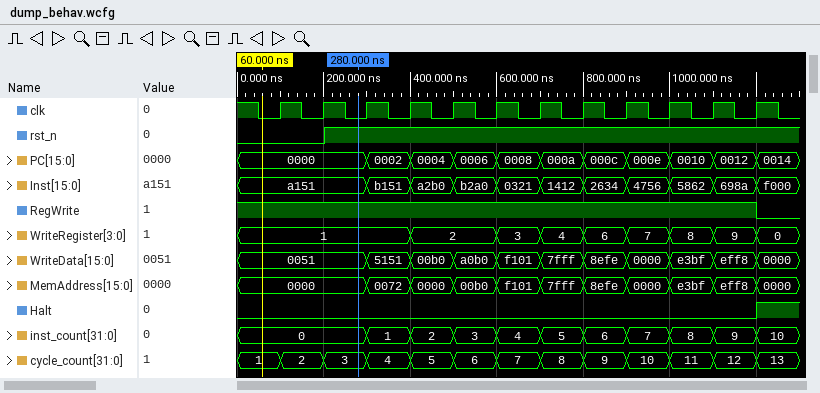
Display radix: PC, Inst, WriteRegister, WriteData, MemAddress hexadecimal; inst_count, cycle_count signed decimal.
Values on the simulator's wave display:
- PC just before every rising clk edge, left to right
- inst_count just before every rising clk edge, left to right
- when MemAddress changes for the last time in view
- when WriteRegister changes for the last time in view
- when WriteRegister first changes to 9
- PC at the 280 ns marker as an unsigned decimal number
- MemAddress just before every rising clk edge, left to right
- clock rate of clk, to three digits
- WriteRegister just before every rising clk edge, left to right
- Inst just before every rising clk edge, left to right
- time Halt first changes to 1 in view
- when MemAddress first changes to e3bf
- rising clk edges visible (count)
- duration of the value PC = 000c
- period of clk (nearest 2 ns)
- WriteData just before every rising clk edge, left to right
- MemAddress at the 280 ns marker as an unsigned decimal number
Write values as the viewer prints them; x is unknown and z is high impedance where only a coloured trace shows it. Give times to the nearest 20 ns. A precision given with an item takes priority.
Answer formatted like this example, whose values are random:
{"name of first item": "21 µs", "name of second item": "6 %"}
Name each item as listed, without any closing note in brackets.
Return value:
{"PC just before every rising clk edge, left to right": "0000, 0000, 0000, 0002, 0004, 0006, 0008, 000a, 000c, 000e, 0010, 0012", "inst_count just before every rising clk edge, left to right": "0, 0, 0, 1, 2, 3, 4, 5, 6, 7, 8, 9", "when MemAddress changes for the last time in view": "1200 ns", "when WriteRegister changes for the last time in view": "1200 ns", "when WriteRegister first changes to 9": "1100 ns", "PC at the 280 ns marker as an unsigned decimal number": "0", "MemAddress just before every rising clk edge, left to right": "0000, 0000, 0000, 0072, 0000, 00b0, f101, 7fff, 8efe, 0000, e3bf, eff8", "clock rate of clk, to three digits": "10.0 MHz", "WriteRegister just before every rising clk edge, left to right": "1, 1, 1, 1, 2, 2, 3, 4, 6, 7, 8, 9", "Inst just before every rising clk edge, left to right": "a151, a151, a151, b151, a2b0, b2a0, 0321, 1412, 2634, 4756, 5862, 698a", "time Halt first changes to 1 in view": "1200 ns", "when MemAddress first changes to e3bf": "1000 ns", "rising clk edges visible": "12", "duration of the value PC = 000c": "100 ns", "period of clk": "100 ns", "WriteData just before every rising clk edge, left to right": "0051, 0051, 0051, 5151, 00b0, a0b0, f101, 7fff, 8efe, 0000, e3bf, eff8", "MemAddress at the 280 ns marker as an unsigned decimal number": "0"}
